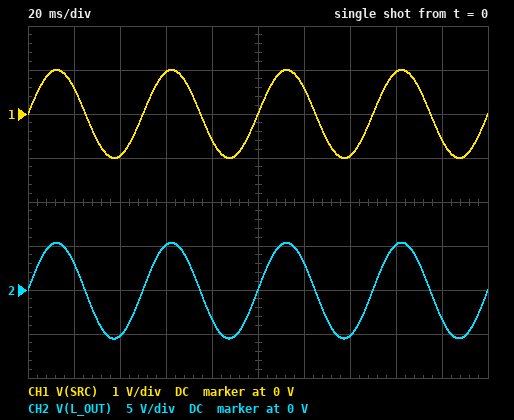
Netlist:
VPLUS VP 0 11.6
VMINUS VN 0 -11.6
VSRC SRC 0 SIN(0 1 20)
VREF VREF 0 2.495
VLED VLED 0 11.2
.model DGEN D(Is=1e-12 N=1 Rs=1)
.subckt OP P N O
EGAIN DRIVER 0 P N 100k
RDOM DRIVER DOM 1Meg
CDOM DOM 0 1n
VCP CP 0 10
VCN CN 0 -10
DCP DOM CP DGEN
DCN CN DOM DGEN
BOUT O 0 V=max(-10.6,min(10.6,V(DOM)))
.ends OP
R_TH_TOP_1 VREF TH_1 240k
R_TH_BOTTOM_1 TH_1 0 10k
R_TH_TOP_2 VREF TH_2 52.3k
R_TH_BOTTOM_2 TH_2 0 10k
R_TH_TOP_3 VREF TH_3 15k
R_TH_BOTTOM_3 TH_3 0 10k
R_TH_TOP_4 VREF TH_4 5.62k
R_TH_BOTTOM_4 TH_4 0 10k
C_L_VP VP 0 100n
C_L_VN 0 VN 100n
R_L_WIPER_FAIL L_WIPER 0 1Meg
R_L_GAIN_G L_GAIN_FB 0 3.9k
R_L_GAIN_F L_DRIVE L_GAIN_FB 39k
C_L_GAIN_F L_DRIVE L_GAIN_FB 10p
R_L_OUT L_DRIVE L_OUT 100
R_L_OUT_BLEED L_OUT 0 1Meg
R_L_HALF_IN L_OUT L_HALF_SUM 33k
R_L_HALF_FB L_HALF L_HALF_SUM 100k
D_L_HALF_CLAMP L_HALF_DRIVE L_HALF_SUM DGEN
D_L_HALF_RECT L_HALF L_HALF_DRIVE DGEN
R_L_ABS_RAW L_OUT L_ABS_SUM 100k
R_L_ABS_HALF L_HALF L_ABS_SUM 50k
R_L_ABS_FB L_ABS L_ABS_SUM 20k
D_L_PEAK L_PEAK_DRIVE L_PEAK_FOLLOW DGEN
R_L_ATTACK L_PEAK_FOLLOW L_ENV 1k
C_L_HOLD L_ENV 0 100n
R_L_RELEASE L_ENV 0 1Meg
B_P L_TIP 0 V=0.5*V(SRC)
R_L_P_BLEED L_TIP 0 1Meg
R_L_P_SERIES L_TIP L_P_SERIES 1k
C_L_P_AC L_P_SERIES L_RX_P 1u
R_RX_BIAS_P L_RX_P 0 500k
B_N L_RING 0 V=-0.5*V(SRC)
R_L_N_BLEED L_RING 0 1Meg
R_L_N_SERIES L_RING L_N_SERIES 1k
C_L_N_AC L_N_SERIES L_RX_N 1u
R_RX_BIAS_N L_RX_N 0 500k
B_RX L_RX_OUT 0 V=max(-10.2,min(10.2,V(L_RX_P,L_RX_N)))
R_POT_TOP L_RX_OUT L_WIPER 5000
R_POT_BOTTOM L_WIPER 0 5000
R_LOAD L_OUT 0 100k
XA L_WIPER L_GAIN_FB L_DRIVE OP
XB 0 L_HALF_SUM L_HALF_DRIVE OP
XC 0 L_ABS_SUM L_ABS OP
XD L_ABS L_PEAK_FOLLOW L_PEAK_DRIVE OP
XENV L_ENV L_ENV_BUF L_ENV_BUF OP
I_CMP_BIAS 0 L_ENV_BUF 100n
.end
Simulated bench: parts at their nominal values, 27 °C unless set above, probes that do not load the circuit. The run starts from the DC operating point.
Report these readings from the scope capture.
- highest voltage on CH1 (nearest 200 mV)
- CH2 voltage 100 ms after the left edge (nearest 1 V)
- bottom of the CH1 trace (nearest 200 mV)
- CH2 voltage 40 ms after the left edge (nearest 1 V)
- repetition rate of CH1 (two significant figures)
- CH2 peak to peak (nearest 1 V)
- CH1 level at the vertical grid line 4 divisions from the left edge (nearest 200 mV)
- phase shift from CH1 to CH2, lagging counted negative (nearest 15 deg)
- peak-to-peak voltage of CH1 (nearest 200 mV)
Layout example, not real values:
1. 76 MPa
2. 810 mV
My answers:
1. 1.0 V
2. 0 V
3. -1.0 V
4. -5 V
5. 20 Hz
6. 11 V
7. -600 mV
8. 0 deg
9. 2.0 V
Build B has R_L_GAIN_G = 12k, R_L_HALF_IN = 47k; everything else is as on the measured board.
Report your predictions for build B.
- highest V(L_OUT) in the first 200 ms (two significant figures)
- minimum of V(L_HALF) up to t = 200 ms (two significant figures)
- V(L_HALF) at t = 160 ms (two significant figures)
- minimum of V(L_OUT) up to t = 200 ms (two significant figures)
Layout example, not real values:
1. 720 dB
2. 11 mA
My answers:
1. 2.1 V
2. -4.4 V
3. -4.2 V
4. -2.1 V
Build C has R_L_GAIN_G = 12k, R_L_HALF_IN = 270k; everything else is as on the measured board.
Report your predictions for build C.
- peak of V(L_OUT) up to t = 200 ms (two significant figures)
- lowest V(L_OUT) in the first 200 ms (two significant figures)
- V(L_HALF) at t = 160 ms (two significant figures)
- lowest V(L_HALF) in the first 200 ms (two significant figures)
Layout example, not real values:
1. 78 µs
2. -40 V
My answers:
1. 2.1 V
2. -2.1 V
3. -740 mV
4. -770 mV
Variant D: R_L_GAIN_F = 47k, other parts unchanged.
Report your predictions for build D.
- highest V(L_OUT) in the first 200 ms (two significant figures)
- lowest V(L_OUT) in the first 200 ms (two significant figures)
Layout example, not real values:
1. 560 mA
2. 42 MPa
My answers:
1. 6.4 V
2. -6.6 V
